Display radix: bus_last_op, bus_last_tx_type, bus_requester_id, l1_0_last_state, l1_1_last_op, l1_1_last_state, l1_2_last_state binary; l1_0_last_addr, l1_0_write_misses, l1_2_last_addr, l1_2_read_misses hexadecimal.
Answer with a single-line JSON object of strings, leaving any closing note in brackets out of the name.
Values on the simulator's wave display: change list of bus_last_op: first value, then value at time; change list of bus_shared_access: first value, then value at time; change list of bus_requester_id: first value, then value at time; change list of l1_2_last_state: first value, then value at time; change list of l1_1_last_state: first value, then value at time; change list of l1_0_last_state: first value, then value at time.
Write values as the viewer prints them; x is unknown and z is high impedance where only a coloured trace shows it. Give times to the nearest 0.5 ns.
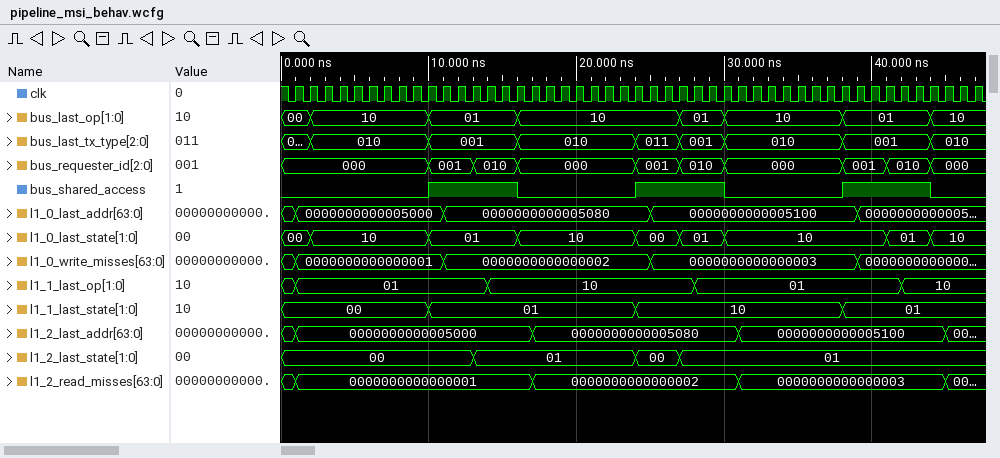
{"change list of bus_last_op: first value, then value at time": "00, 10 at 2 ns, 01 at 10 ns, 10 at 16 ns, 01 at 27 ns, 10 at 30 ns, 01 at 38 ns, 10 at 44 ns", "change list of bus_shared_access: first value, then value at time": "0, 1 at 10 ns, 0 at 16 ns, 1 at 24 ns, 0 at 30 ns, 1 at 38 ns, 0 at 44 ns", "change list of bus_requester_id: first value, then value at time": "000, 001 at 10 ns, 010 at 13 ns, 000 at 16 ns, 001 at 24 ns, 010 at 27 ns, 000 at 30 ns, 001 at 38 ns, 010 at 41 ns, 000 at 44 ns", "change list of l1_2_last_state: first value, then value at time": "00, 01 at 13 ns, 00 at 24 ns, 01 at 27 ns", "change list of l1_1_last_state: first value, then value at time": "00, 01 at 10 ns, 10 at 24 ns, 01 at 38 ns", "change list of l1_0_last_state: first value, then value at time": "00, 10 at 2 ns, 01 at 10 ns, 10 at 16 ns, 00 at 24 ns, 01 at 27 ns, 10 at 30 ns, 01 at 41 ns, 10 at 44 ns"}
